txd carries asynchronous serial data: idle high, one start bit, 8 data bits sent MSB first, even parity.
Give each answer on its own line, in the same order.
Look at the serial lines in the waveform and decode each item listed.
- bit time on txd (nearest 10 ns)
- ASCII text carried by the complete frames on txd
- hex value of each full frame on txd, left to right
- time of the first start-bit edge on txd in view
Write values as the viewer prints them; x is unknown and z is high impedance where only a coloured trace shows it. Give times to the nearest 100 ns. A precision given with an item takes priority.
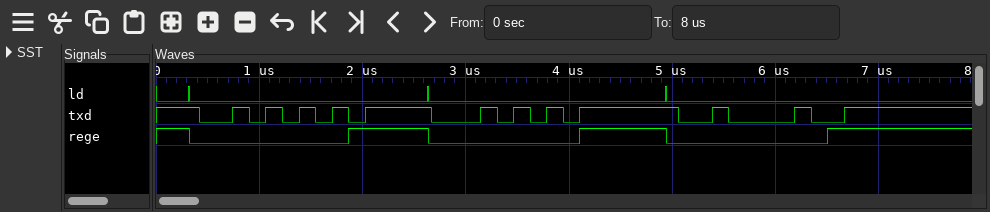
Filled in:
160 ns
"U*B"
55, 2A, 42
400 ns
